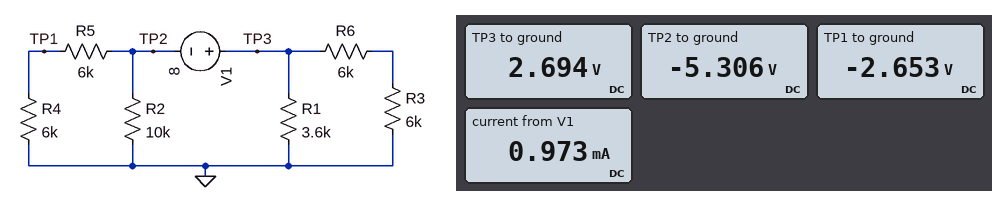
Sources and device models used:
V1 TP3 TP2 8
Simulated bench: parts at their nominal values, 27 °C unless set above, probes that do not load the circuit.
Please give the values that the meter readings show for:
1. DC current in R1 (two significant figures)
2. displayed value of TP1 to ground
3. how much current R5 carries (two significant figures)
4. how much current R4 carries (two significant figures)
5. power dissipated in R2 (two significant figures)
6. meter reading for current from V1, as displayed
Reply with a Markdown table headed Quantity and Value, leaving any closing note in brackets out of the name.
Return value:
| Quantity | Value |
|---|---|
| DC current in R1 | 750 µA |
| displayed value of TP1 to ground | -2.653 V |
| how much current R5 carries | 440 µA |
| how much current R4 carries | 440 µA |
| power dissipated in R2 | 2.8 mW |
| meter reading for current from V1, as displayed | 0.973 mA |
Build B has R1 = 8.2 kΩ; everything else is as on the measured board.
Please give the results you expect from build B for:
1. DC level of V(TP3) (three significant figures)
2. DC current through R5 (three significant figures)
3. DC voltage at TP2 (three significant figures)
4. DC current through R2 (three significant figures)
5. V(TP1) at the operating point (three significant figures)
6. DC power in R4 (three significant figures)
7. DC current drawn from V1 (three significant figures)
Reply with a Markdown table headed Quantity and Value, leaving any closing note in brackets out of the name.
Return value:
| Quantity | Value |
|---|---|
| DC level of V(TP3) | 3.77 V |
| DC current through R5 | 352 µA |
| DC voltage at TP2 | -4.23 V |
| DC current through R2 | 423 µA |
| V(TP1) at the operating point | -2.11 V |
| DC power in R4 | 744 µW |
| DC current drawn from V1 | 775 µA |
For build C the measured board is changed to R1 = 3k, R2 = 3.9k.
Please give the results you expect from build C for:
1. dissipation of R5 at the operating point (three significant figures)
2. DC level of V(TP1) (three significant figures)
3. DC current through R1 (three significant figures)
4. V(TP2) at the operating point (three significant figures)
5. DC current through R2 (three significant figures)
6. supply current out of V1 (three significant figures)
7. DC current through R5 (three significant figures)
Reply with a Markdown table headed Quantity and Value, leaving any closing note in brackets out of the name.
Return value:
| Quantity | Value |
|---|---|
| dissipation of R5 at the operating point | 809 µW |
| DC level of V(TP1) | -2.20 V |
| DC current through R1 | 1.20 mA |
| V(TP2) at the operating point | -4.41 V |
| DC current through R2 | 1.13 mA |
| supply current out of V1 | 1.50 mA |
| DC current through R5 | 367 µA |
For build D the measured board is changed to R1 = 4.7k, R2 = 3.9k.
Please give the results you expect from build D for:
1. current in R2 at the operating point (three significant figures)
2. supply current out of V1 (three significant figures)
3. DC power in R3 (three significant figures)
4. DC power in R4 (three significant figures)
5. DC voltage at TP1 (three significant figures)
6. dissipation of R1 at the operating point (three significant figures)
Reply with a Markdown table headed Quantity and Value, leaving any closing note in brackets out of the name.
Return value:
| Quantity | Value |
|---|---|
| current in R2 at the operating point | 955 µA |
| supply current out of V1 | 1.27 mA |
| DC power in R3 | 761 µW |
| DC power in R4 | 578 µW |
| DC voltage at TP1 | -1.86 V |
| dissipation of R1 at the operating point | 3.89 mW |
